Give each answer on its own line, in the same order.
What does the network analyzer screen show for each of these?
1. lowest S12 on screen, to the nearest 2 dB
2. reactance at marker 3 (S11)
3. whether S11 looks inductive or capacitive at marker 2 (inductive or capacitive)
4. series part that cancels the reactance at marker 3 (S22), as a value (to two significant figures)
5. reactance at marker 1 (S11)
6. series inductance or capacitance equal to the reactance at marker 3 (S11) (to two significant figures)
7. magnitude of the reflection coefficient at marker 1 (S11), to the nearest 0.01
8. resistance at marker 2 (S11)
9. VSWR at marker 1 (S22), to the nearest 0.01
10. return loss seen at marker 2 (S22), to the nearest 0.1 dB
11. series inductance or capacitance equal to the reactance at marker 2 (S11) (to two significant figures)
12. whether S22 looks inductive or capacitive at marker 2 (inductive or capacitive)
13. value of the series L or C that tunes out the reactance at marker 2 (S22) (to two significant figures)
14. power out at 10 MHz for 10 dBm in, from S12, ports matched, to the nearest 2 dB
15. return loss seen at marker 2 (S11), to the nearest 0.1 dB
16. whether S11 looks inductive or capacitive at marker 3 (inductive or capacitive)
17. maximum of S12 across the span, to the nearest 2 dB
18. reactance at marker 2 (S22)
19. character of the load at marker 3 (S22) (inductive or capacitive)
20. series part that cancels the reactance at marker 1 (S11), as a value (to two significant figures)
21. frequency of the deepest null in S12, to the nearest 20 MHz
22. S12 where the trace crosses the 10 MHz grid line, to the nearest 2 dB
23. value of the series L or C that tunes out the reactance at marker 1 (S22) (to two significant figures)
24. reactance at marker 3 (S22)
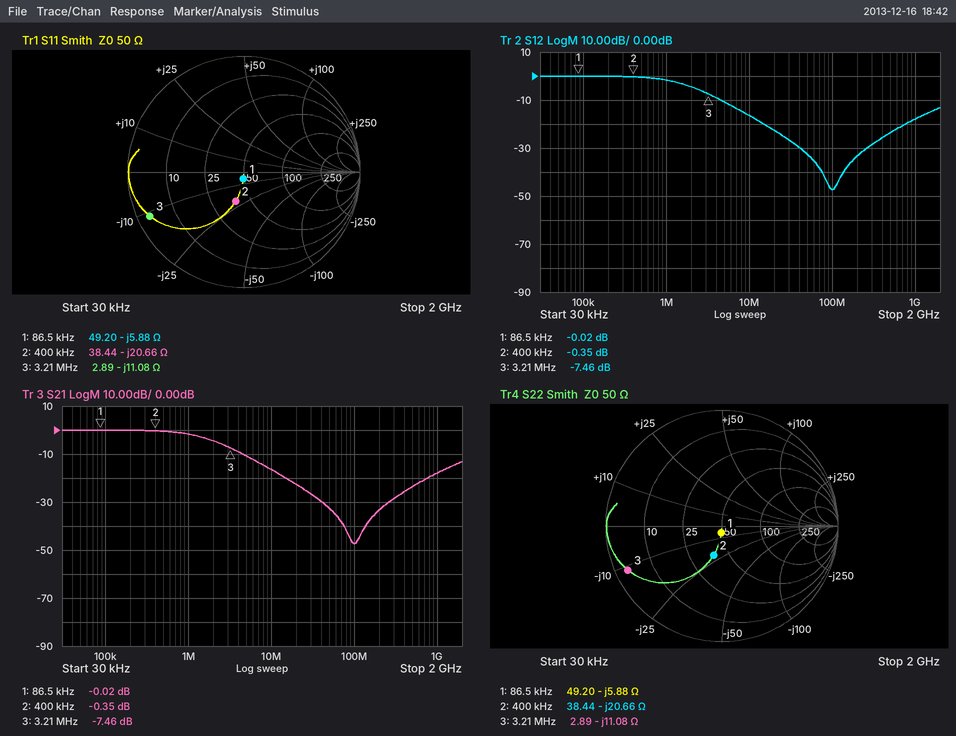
-48 dB
-11.08 Ω
capacitive
550 nH
-5.88 Ω
4.5 nF
0.06
38.44 Ω
1.13
11.7 dB
19 nF
capacitive
8.2 µH
-6 dBm
11.7 dB
capacitive
0 dB
-20.66 Ω
capacitive
11 µH
100 MHz
-16 dB
11 µH
-11.08 Ω
